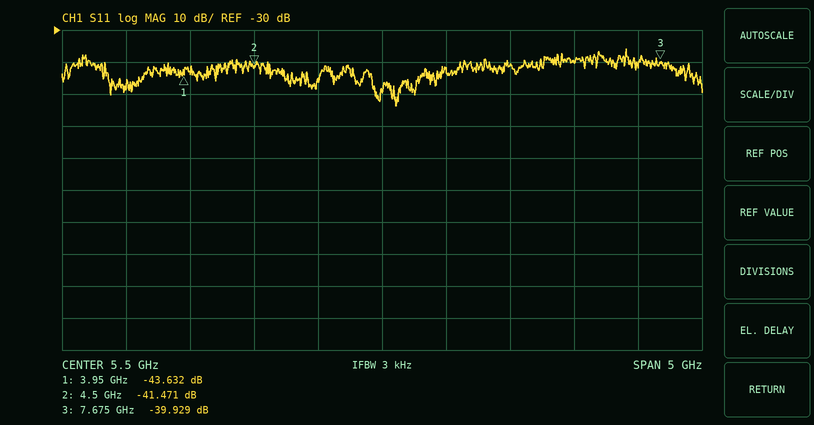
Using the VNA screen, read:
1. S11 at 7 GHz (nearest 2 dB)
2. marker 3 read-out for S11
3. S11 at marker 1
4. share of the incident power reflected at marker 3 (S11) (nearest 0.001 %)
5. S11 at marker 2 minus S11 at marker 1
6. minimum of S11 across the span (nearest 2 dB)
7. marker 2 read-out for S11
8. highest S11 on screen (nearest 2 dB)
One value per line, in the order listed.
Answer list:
-40 dB
-39.929 dB
-43.632 dB
0.010 %
2.161 dB
-54 dB
-41.471 dB
-36 dB
